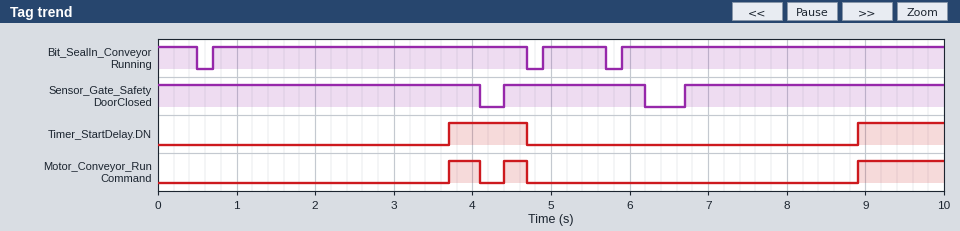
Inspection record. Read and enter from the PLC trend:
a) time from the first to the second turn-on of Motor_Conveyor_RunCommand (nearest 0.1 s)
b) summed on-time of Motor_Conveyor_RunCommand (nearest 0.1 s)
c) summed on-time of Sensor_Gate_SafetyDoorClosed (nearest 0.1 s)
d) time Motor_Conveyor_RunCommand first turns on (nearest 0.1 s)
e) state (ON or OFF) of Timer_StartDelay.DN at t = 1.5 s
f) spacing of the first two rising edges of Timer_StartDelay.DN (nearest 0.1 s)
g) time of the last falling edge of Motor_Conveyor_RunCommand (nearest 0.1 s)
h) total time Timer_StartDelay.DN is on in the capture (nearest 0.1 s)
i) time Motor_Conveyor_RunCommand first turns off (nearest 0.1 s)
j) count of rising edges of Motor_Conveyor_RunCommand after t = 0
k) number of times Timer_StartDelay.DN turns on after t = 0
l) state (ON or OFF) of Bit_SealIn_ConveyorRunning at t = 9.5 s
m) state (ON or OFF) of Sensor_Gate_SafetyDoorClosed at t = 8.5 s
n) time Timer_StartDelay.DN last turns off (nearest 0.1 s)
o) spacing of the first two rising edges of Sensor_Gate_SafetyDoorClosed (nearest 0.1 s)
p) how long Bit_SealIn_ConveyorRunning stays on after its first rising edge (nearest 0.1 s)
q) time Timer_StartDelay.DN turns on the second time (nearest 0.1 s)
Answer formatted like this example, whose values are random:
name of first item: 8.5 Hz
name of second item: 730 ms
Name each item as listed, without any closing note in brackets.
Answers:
time from the first to the second turn-on of Motor_Conveyor_RunCommand: 0.7 s
summed on-time of Motor_Conveyor_RunCommand: 1.8 s
summed on-time of Sensor_Gate_SafetyDoorClosed: 9.2 s
time Motor_Conveyor_RunCommand first turns on: 3.7 s
state (ON or OFF) of Timer_StartDelay.DN at t = 1.5 s: OFF
spacing of the first two rising edges of Timer_StartDelay.DN: 5.2 s
time of the last falling edge of Motor_Conveyor_RunCommand: 4.7 s
total time Timer_StartDelay.DN is on in the capture: 2.1 s
time Motor_Conveyor_RunCommand first turns off: 4.1 s
count of rising edges of Motor_Conveyor_RunCommand after t = 0: 3
number of times Timer_StartDelay.DN turns on after t = 0: 2
state (ON or OFF) of Bit_SealIn_ConveyorRunning at t = 9.5 s: ON
state (ON or OFF) of Sensor_Gate_SafetyDoorClosed at t = 8.5 s: ON
time Timer_StartDelay.DN last turns off: 4.7 s
spacing of the first two rising edges of Sensor_Gate_SafetyDoorClosed: 2.3 s
how long Bit_SealIn_ConveyorRunning stays on after its first rising edge: 4.0 s
time Timer_StartDelay.DN turns on the second time: 8.9 s
